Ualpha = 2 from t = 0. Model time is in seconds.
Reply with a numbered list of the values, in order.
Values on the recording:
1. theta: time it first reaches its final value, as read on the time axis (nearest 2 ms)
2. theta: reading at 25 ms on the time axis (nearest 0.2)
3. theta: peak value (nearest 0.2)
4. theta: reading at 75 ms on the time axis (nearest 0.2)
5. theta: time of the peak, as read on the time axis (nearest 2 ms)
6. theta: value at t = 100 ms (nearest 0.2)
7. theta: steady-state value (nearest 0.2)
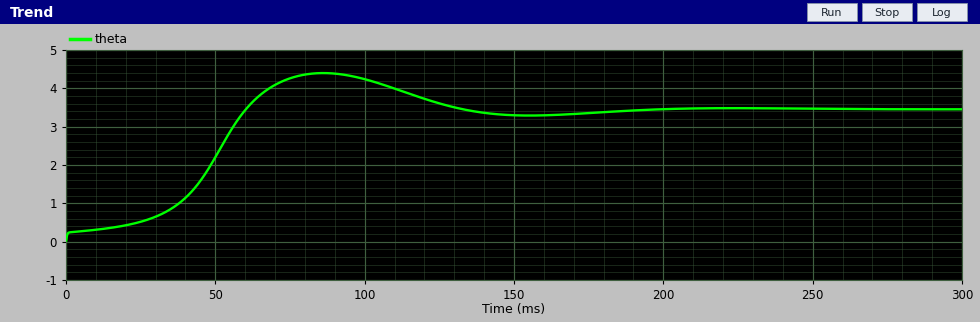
1. 60 ms
2. 0.6
3. 4.4
4. 4.2
5. 86 ms
6. 4.2
7. 3.4
